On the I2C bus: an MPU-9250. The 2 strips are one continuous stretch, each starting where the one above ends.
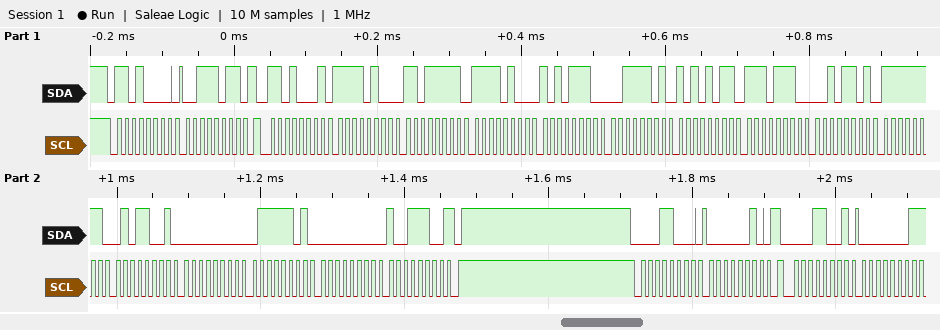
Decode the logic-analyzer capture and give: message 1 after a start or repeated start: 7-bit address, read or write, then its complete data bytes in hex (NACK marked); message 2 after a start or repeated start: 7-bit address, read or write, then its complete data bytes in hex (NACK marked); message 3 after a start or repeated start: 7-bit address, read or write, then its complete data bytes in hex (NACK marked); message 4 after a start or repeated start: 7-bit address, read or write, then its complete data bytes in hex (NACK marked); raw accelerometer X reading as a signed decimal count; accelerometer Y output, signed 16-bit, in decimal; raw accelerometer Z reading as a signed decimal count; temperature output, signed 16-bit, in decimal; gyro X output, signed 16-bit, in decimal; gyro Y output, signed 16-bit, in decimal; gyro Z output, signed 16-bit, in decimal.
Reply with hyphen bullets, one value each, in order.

- 0x68 write: 3B
- 0x68 read: F4 DF F4 AE 3D AB EE 2D FF 59 00 7D 00 9C NACK
- 0x0C write: 02
- 0x0C read: 01 NACK
- -2849
- -2898
- 15787
- -4563
- -167
- 125
- 156
